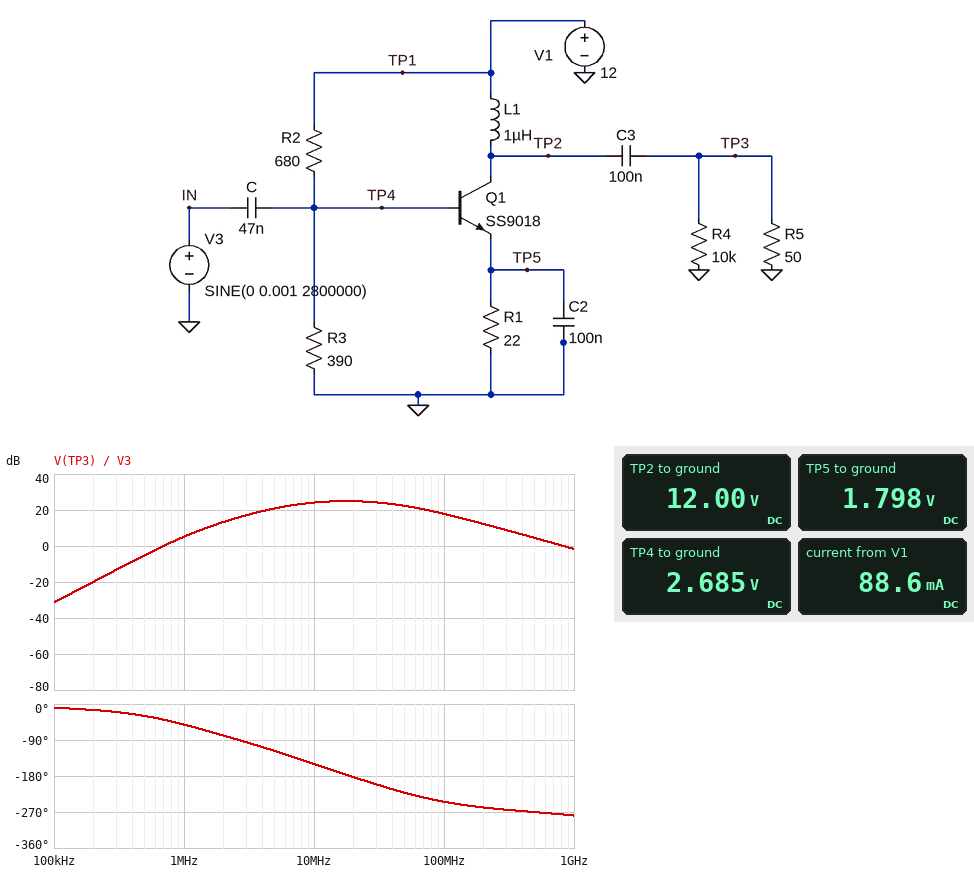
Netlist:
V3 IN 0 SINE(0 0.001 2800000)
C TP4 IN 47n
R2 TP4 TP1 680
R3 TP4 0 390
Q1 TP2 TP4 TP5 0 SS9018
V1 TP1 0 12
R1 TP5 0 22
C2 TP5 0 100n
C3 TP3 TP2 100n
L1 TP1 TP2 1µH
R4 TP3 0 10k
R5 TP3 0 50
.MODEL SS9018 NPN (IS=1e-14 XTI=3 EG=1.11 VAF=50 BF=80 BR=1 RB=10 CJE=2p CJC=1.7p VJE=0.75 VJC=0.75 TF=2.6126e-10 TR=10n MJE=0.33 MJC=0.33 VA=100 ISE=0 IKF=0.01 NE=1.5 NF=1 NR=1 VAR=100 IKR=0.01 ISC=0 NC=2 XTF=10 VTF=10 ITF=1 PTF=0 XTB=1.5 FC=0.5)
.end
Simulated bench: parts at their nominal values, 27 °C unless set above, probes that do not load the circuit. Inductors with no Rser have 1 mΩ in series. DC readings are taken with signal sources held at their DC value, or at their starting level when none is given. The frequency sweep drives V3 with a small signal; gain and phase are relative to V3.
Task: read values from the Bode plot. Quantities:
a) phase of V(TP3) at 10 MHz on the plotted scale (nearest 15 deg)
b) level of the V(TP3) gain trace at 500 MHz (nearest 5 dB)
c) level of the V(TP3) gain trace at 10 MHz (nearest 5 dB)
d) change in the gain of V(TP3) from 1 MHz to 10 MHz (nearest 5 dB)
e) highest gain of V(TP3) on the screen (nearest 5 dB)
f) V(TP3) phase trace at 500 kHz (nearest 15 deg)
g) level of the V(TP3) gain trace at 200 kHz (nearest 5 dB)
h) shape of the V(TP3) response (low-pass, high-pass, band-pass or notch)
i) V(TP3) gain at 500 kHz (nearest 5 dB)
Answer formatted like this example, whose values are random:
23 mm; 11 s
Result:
-150 deg; 5 dB; 25 dB; 20 dB; 25 dB; -30 deg; -20 dB; band-pass; -5 dB
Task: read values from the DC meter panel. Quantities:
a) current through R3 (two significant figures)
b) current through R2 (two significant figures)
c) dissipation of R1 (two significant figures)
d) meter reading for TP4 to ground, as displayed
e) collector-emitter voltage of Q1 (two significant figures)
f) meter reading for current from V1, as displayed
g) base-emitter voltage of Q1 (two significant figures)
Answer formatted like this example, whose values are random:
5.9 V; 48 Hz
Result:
6.9 mA; 14 mA; 150 mW; 2.685 V; 10 V; 88.6 mA; 890 mV
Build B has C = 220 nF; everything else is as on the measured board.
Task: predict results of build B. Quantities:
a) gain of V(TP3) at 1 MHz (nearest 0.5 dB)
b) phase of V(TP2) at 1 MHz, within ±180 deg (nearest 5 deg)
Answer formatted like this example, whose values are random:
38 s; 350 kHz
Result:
6.0 dB; -60 deg
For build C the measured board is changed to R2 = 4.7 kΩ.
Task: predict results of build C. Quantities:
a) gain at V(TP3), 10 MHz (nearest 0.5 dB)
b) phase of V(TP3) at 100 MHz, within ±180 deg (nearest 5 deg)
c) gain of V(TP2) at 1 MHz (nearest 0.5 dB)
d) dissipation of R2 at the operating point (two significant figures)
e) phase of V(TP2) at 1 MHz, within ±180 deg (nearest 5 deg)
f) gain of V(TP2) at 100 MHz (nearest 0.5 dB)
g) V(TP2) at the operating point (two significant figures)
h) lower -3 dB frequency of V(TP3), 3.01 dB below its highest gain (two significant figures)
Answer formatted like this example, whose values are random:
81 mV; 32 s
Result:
17.0 dB; 165 deg; 0.5 dB; 26 mW; -80 deg; 18.5 dB; 12 V; 7.5 MHz
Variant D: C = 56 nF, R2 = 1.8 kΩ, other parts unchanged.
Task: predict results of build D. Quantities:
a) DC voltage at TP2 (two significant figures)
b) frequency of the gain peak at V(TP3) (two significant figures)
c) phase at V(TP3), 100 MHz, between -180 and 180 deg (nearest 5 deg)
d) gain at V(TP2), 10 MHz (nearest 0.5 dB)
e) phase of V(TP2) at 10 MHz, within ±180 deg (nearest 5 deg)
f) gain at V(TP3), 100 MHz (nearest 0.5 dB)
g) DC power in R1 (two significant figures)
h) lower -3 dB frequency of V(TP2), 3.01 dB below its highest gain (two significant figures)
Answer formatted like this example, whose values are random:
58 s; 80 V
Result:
12 V; 27 MHz; 135 deg; 25.0 dB; -145 deg; 24.0 dB; 29 mW; 6.9 MHz
